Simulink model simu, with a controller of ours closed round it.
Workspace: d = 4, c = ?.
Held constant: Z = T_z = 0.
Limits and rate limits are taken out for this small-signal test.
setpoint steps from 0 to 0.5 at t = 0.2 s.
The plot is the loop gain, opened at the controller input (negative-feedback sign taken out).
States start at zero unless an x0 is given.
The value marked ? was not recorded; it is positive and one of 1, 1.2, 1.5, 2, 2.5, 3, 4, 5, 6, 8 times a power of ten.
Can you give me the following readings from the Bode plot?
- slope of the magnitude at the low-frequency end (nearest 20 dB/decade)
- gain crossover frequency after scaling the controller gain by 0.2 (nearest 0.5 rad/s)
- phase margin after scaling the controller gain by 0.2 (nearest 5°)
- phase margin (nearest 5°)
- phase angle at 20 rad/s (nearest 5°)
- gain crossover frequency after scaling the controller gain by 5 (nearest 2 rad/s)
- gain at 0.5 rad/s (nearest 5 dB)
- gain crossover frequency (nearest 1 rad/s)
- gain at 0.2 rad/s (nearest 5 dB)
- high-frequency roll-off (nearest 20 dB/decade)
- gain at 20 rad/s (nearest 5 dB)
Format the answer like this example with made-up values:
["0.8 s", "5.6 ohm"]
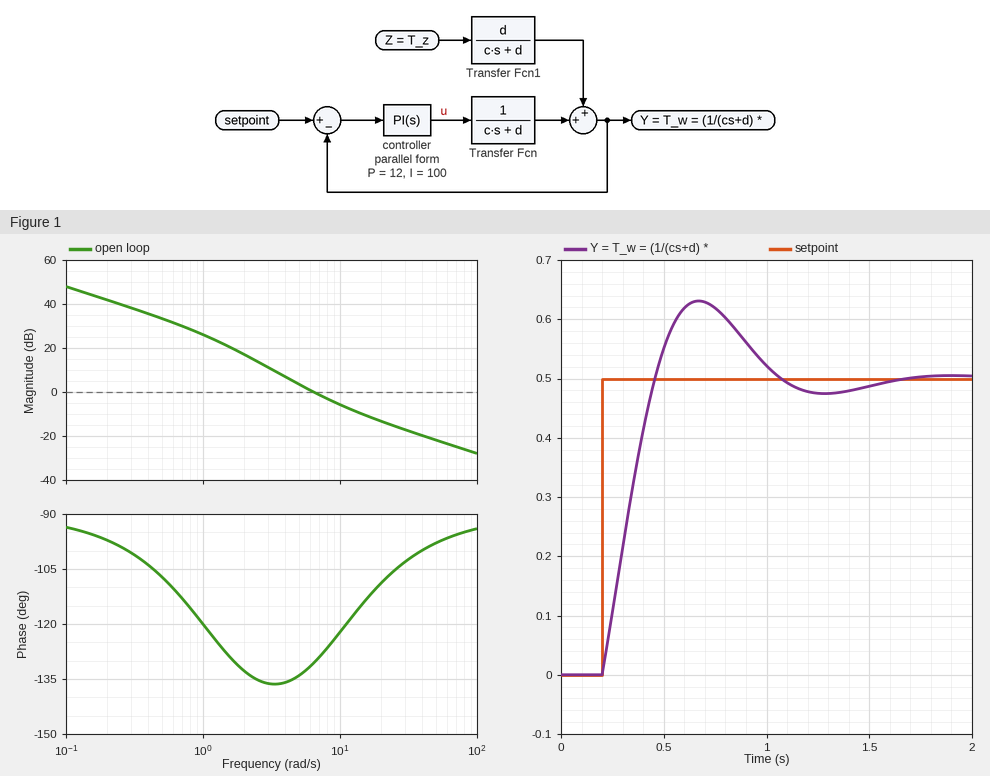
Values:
["-20 dB/decade", "2.5 rad/s", "45°", "50°", "-110°", "22 rad/s", "35 dB", "6 rad/s", "40 dB", "-20 dB/decade", "-15 dB"]
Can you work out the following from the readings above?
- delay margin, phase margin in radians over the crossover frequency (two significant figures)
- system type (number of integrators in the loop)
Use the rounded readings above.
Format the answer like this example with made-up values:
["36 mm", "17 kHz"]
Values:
["0.15 s", "1"]
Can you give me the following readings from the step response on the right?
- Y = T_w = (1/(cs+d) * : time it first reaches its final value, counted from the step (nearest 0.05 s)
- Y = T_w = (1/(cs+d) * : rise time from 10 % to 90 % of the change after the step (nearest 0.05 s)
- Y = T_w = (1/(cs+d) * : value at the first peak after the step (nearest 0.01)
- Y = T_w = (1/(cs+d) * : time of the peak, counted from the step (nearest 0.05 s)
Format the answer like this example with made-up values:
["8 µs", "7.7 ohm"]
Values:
["0.25 s", "0.20 s", "0.63", "0.45 s"]
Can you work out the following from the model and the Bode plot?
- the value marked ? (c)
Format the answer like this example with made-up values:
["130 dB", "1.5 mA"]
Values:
["3"]
